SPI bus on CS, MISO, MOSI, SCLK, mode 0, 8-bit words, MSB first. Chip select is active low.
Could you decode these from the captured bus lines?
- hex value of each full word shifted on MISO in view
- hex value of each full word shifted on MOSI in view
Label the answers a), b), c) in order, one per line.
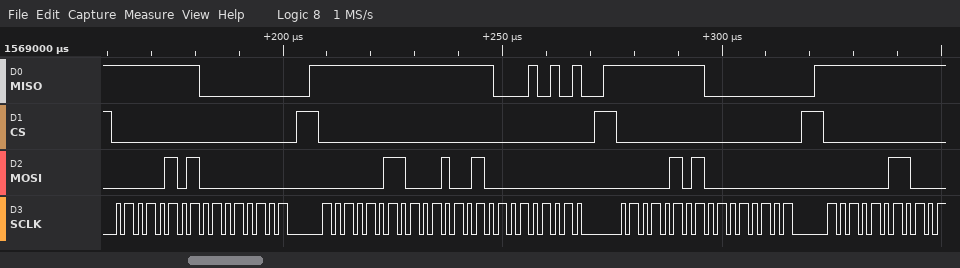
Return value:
a) FF, 00, FF, FF, 15, FF, 00, FF
b) 05, 00, 03, 12, 00, 05, 00, 03
